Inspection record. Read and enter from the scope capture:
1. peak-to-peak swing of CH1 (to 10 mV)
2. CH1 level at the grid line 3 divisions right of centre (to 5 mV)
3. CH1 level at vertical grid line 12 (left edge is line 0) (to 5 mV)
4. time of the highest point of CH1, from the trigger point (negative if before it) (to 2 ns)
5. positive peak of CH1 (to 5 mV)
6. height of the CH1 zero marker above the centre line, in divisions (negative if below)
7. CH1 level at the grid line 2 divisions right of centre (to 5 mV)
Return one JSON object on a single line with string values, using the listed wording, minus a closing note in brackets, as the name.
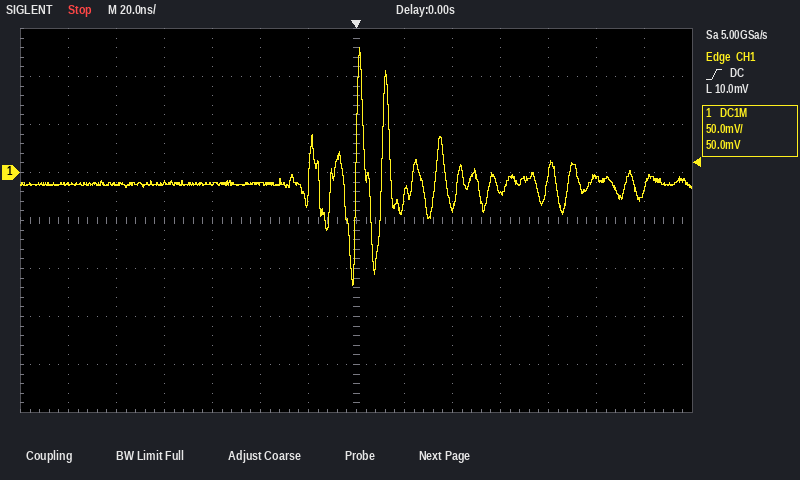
{"peak-to-peak swing of CH1": "250 mV", "CH1 level at the grid line 3 divisions right of centre": "-20 mV", "CH1 level at vertical grid line 12 (left edge is line 0)": "-5 mV", "time of the highest point of CH1, from the trigger point (negative if before it)": "+2 ns", "positive peak of CH1": "130 mV", "height of the CH1 zero marker above the centre line, in divisions": "+1.0 div", "CH1 level at the grid line 2 divisions right of centre": "-35 mV"}
